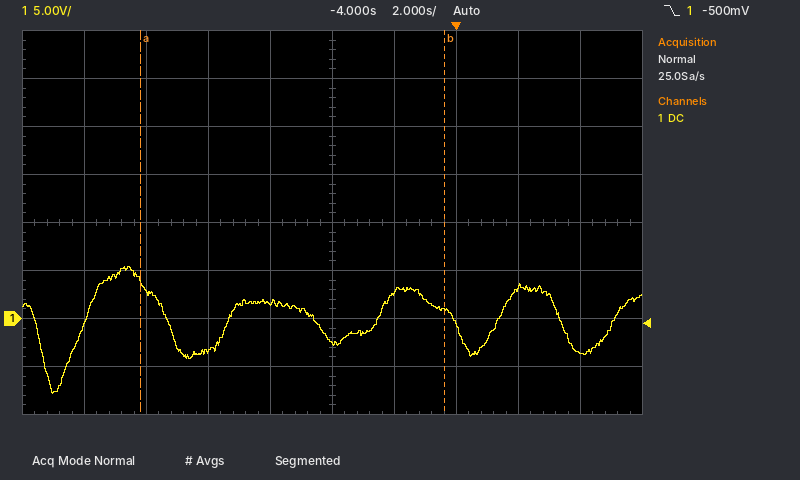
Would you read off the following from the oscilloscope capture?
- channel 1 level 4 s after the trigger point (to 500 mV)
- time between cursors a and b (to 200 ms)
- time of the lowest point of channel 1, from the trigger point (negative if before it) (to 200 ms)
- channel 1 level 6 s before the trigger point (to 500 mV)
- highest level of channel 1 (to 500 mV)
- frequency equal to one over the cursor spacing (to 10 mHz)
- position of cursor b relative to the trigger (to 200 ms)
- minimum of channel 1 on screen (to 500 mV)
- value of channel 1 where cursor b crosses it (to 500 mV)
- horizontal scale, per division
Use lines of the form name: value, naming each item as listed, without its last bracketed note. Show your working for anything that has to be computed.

channel 1 level 4 s after the trigger point: -3.5 V
time between cursors a and b: 9.8 s
time of the lowest point of channel 1, from the trigger point (negative if before it): -13.0 s
channel 1 level 6 s before the trigger point: 1.5 V
highest level of channel 1: 5.5 V
frequency equal to one over the cursor spacing: 1 / 9.8 s ≈ 100 mHz
position of cursor b relative to the trigger: -400 ms
minimum of channel 1 on screen: -8.0 V
value of channel 1 where cursor b crosses it: 1.0 V
horizontal scale, per division: 2 s
